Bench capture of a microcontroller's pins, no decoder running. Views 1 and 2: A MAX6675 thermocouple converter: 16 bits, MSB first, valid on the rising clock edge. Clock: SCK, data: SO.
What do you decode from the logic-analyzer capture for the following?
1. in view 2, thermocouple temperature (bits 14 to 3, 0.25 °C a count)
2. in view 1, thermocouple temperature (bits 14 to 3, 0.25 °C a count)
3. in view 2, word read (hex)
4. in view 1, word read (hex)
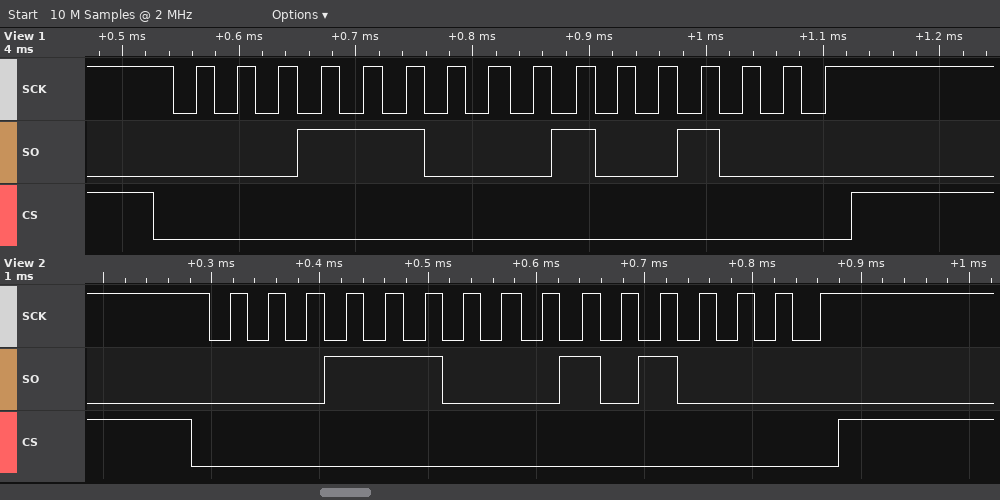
226.50 °C
226.25 °C
0x1C50
0x1C48
